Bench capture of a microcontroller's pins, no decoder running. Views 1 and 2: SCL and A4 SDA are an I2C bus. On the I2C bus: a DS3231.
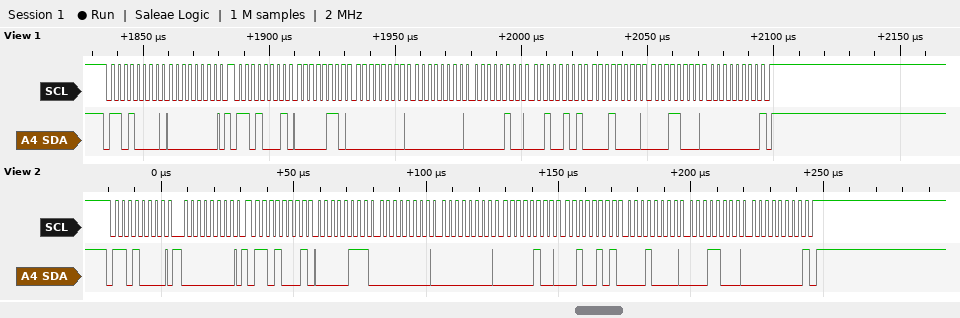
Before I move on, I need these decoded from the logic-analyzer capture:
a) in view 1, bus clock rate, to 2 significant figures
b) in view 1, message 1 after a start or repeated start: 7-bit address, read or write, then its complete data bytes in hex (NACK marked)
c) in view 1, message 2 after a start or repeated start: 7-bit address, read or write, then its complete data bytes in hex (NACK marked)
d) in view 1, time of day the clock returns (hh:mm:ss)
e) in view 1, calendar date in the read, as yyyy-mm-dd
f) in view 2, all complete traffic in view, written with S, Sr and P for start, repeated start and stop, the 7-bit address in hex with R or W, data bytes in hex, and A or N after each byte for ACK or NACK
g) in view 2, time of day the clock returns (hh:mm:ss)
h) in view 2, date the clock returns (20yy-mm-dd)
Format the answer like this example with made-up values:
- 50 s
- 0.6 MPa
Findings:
- 400 kHz
- 0x68 write: 00
- 0x68 read: 06 00 00 04 25 10 18 00 NACK
- 00:00:06
- 2018-10-25
- S 68W A 00 A Sr 68R A 07 A 00 A 00 A 04 A 25 A 10 A 18 A 00 N P
- 00:00:07
- 2018-10-25
